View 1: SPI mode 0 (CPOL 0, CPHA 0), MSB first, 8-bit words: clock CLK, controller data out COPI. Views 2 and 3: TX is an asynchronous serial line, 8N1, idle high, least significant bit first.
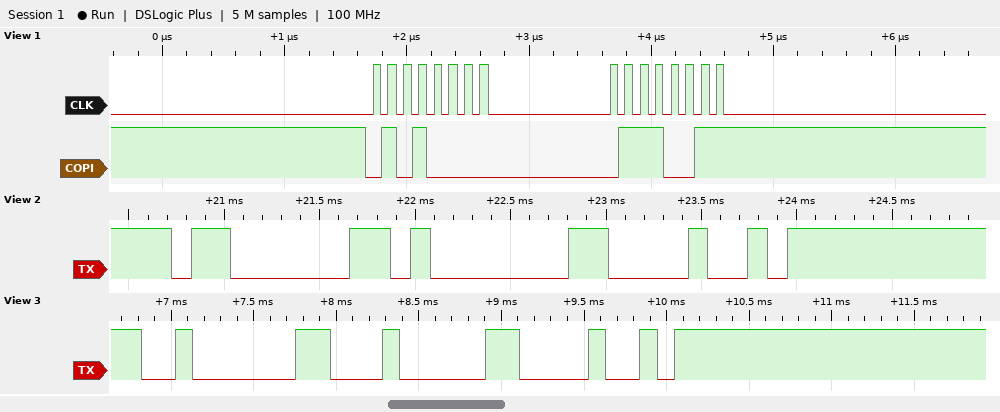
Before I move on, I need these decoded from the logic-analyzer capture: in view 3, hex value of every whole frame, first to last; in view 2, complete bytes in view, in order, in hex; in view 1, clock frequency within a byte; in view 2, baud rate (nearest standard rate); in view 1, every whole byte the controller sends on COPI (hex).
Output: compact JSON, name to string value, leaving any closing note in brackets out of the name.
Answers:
{"in view 3, hex value of every whole frame, first to last": "02 04 48", "in view 2, complete bytes in view, in order, in hex": "03 01 48", "in view 1, clock frequency within a byte": "8 MHz", "in view 2, baud rate": "9600 baud", "in view 1, every whole byte the controller sends on COPI": "0x50 0x73"}
